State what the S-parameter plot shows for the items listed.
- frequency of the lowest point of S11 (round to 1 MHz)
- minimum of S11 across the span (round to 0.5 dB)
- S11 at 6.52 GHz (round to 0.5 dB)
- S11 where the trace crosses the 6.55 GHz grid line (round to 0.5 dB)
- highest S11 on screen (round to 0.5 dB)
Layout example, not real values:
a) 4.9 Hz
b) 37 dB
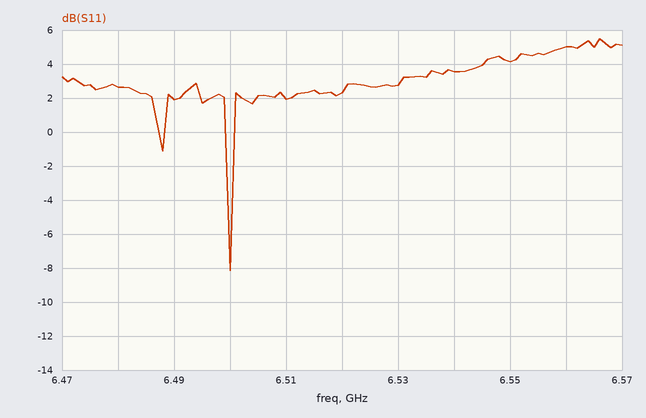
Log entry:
a) 6.500 GHz
b) -8.0 dB
c) 2.5 dB
d) 4.0 dB
e) 5.5 dB
